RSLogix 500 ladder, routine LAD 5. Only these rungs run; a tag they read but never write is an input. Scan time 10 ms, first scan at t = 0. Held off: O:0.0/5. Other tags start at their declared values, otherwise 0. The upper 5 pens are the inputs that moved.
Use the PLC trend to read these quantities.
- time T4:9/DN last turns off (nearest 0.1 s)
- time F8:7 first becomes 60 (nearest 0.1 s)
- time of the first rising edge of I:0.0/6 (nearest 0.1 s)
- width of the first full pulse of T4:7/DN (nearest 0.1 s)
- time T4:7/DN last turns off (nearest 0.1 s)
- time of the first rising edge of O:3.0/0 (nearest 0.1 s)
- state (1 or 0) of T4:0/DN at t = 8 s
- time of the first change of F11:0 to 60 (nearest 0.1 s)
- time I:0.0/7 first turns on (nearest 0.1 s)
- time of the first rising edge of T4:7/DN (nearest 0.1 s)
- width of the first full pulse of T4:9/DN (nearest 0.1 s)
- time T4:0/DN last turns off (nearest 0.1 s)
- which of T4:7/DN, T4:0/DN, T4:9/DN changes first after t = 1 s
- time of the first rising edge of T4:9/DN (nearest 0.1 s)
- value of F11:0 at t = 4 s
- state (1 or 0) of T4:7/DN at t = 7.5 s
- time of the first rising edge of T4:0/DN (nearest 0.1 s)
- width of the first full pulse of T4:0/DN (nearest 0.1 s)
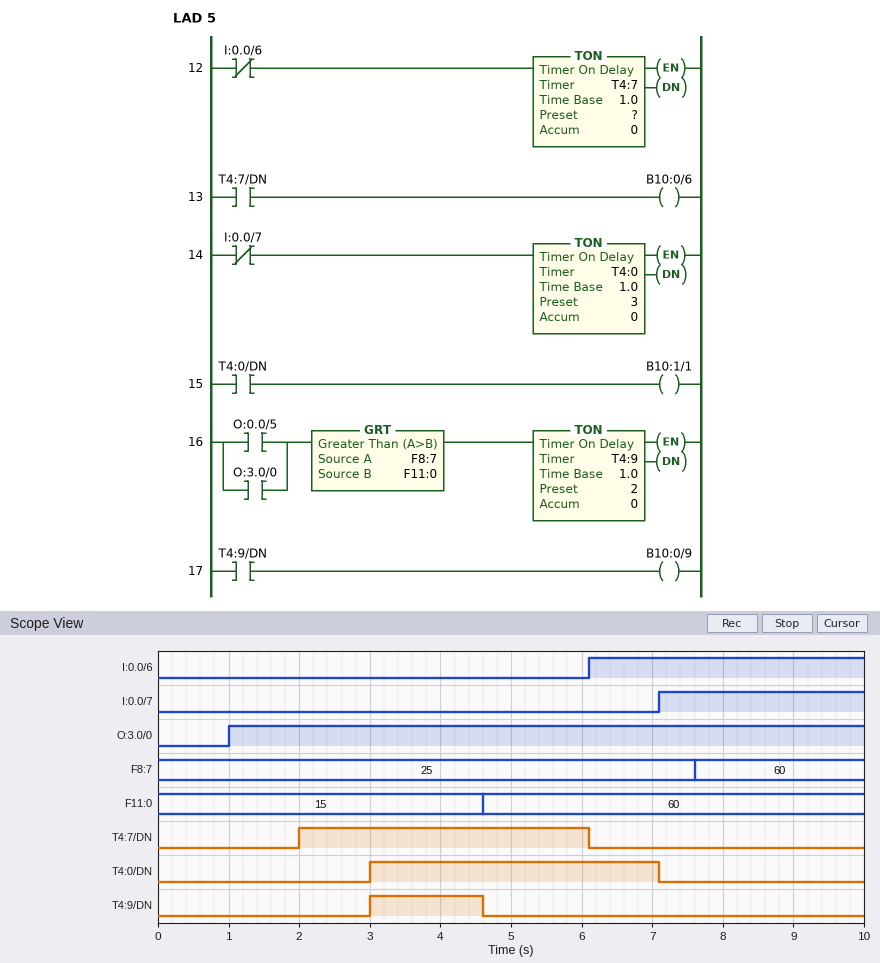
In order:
4.6 s
7.6 s
6.1 s
4.1 s
6.1 s
1.0 s
0
4.6 s
7.1 s
2.0 s
1.6 s
7.1 s
T4:7/DN
3.0 s
15
0
3.0 s
4.1 s
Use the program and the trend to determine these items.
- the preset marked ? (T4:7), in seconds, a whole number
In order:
2 s
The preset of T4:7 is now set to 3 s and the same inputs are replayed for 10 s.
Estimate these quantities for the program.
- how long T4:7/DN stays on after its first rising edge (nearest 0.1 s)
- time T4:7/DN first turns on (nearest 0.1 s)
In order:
3.1 s
3.0 s
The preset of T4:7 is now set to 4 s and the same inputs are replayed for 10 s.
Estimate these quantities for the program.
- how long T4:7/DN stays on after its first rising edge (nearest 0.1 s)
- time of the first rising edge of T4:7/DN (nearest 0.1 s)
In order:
2.1 s
4.0 s
